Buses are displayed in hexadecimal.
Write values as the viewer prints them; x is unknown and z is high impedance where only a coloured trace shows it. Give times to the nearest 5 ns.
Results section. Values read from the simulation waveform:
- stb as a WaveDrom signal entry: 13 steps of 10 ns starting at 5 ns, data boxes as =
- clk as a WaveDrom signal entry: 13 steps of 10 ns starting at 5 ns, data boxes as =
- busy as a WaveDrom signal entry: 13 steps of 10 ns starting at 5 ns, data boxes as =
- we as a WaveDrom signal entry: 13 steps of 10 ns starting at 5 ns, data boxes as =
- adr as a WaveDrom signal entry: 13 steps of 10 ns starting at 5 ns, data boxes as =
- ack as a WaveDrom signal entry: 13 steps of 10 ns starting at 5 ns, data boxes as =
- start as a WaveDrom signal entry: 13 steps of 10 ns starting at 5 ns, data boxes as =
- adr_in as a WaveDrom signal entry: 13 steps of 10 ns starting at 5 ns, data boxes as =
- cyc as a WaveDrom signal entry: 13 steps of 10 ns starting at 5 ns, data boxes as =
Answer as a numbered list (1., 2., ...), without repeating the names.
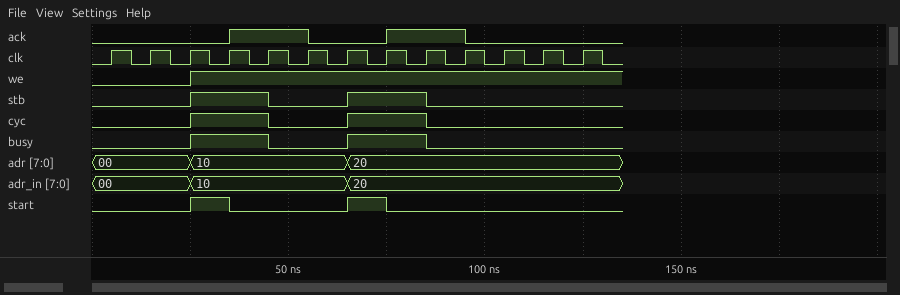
1. {name: 'stb', wave: '0.1.0.1.0....'}
2. {name: 'clk', wave: 'p............'}
3. {name: 'busy', wave: '0.1.0.1.0....'}
4. {name: 'we', wave: '0.1..........'}
5. {name: 'adr', wave: '=.=...=......', data: '00 10 20'}
6. {name: 'ack', wave: '0..1.0.1.0...'}
7. {name: 'start', wave: '0.10..10.....'}
8. {name: 'adr_in', wave: '=.=...=......', data: '00 10 20'}
9. {name: 'cyc', wave: '0.1.0.1.0....'}
